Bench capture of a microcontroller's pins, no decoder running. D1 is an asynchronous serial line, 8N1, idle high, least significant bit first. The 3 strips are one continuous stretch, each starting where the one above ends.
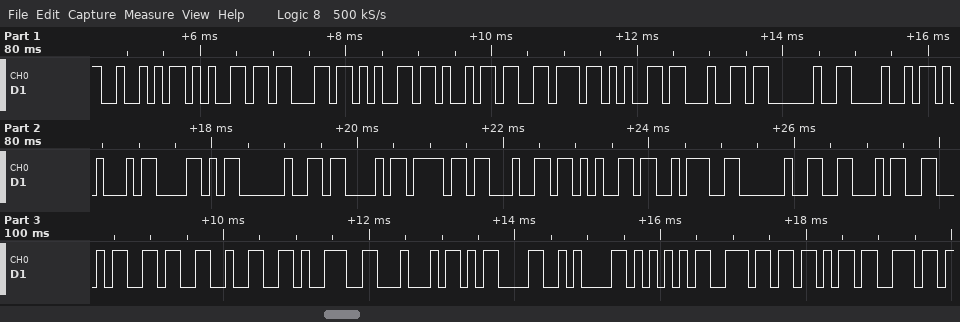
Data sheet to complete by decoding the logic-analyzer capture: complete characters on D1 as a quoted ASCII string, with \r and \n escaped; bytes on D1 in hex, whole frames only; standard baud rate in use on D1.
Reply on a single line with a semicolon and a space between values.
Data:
"Received HEX Code: FF629D\r\nUnkn"; 52 65 63 65 69 76 65 64 20 48 45 58 20 43 6F 64 65 3A 20 46 46 36 32 39 44 0D 0A 55 6E 6B 6E; 9600 baud
